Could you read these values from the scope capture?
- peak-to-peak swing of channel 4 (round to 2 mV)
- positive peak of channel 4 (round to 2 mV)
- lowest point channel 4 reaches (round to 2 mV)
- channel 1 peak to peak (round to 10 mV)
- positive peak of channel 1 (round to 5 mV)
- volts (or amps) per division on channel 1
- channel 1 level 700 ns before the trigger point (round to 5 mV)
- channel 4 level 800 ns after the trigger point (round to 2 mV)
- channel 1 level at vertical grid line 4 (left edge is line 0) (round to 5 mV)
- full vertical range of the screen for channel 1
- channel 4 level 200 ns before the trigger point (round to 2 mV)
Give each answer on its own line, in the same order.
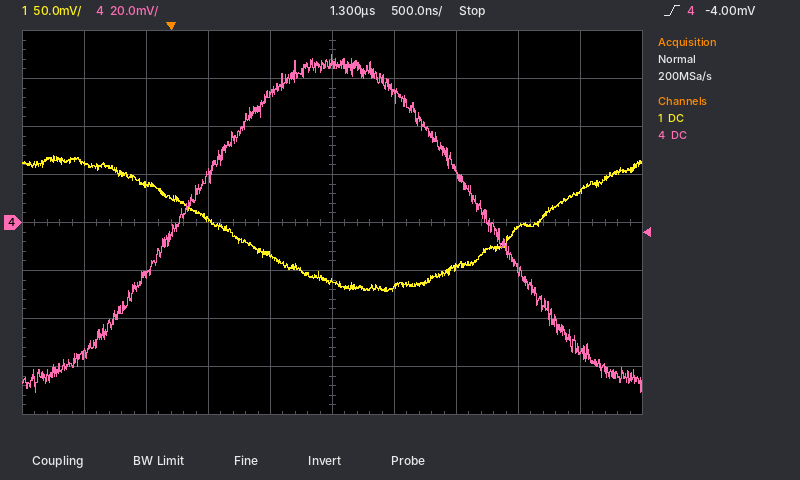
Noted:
140 mV
70 mV
-70 mV
140 mV
70 mV
50 mV
60 mV
54 mV
-35 mV
400 mV
-22 mV
